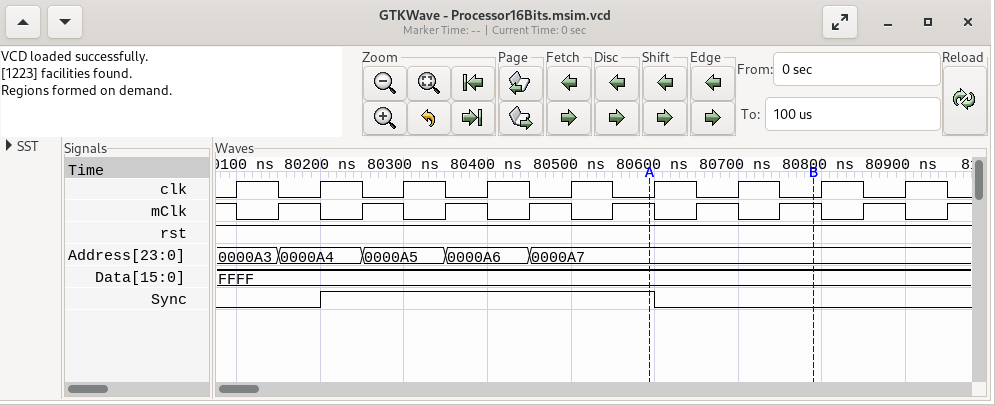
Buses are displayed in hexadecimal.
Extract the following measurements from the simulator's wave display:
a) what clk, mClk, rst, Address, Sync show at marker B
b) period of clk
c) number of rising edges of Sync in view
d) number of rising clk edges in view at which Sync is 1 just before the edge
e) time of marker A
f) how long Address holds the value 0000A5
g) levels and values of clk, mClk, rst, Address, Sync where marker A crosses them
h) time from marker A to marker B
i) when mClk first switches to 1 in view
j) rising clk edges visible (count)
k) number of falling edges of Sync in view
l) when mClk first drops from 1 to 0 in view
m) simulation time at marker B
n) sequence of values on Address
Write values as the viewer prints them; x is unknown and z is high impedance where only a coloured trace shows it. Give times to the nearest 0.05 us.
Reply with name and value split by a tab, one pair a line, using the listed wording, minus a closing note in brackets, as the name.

what clk, mClk, rst, Address, Sync show at marker B	clk=0, mClk=1, rst=1, Address=0000A7, Sync=0
period of clk	0.1 us
number of rising edges of Sync in view	1
number of rising clk edges in view at which Sync is 1 just before the edge	4
time of marker A	80.6 us
how long Address holds the value 0000A5	0.1 us
levels and values of clk, mClk, rst, Address, Sync where marker A crosses them	clk=0, mClk=1, rst=1, Address=0000A7, Sync=1
time from marker A to marker B	0.2 us
when mClk first switches to 1 in view	80.15 us
rising clk edges visible	9
number of falling edges of Sync in view	1
when mClk first drops from 1 to 0 in view	80.1 us
simulation time at marker B	80.8 us
sequence of values on Address	0000A3, 0000A4, 0000A5, 0000A6, 0000A7
